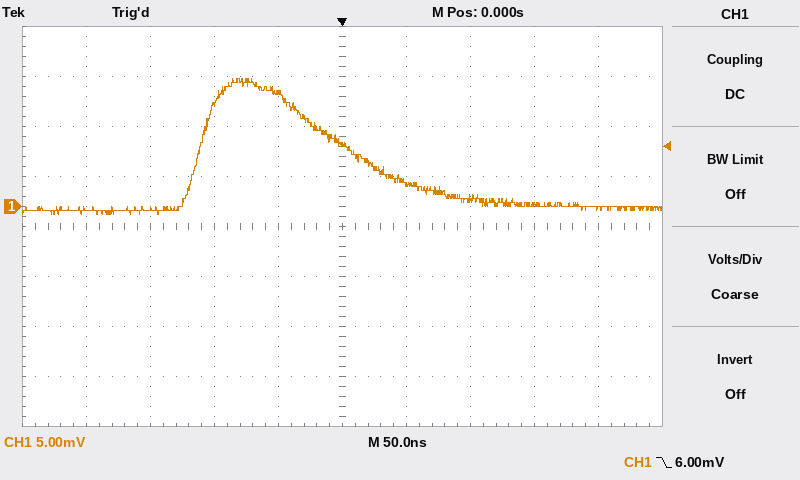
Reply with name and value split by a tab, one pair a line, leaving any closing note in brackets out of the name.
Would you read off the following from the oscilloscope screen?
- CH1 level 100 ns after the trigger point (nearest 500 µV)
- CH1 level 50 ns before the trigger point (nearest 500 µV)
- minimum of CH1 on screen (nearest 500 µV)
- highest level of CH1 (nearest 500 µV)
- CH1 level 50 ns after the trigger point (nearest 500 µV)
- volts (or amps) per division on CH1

CH1 level 100 ns after the trigger point	1.0 mV
CH1 level 50 ns before the trigger point	11.5 mV
minimum of CH1 on screen	-1.0 mV
highest level of CH1	13.0 mV
CH1 level 50 ns after the trigger point	2.5 mV
volts (or amps) per division on CH1	5 mV
